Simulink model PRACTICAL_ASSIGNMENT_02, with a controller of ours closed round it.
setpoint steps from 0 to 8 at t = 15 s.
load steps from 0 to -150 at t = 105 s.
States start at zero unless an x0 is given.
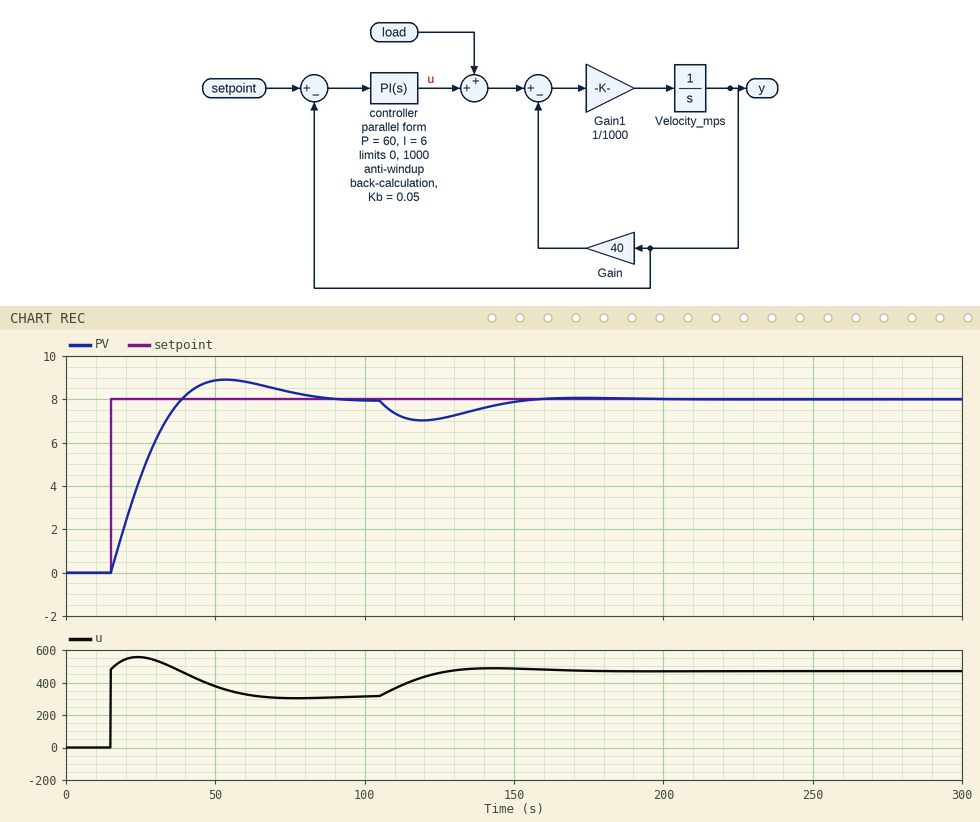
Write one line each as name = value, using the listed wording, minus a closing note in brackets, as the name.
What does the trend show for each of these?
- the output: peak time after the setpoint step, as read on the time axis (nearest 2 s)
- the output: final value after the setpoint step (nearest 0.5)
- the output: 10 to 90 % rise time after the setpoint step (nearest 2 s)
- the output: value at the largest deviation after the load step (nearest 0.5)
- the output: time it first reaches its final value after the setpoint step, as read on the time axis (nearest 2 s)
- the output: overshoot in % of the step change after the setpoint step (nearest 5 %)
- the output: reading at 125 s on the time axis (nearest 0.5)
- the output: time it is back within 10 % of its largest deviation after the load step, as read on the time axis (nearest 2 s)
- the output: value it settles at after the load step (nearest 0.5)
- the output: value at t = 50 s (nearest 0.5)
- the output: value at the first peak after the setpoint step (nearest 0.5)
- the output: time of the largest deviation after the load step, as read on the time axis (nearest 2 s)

the output: peak time after the setpoint step, as read on the time axis = 54 s
the output: final value after the setpoint step = 8.0
the output: 10 to 90 % rise time after the setpoint step = 18 s
the output: value at the largest deviation after the load step = 7.0
the output: time it first reaches its final value after the setpoint step, as read on the time axis = 38 s
the output: overshoot in % of the step change after the setpoint step = 10 %
the output: reading at 125 s on the time axis = 7.0
the output: time it is back within 10 % of its largest deviation after the load step, as read on the time axis = 152 s
the output: value it settles at after the load step = 8.0
the output: value at t = 50 s = 9.0
the output: value at the first peak after the setpoint step = 9.0
the output: time of the largest deviation after the load step, as read on the time axis = 120 s
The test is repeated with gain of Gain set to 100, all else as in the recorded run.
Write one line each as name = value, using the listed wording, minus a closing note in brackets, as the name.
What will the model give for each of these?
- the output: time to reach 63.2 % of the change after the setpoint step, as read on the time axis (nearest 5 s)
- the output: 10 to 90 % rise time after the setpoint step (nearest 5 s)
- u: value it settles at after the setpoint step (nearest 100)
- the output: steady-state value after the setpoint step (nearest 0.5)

the output: time to reach 63.2 % of the change after the setpoint step, as read on the time axis = 30 s
the output: 10 to 90 % rise time after the setpoint step = 35 s
u: value it settles at after the setpoint step = 800
the output: steady-state value after the setpoint step = 8.0
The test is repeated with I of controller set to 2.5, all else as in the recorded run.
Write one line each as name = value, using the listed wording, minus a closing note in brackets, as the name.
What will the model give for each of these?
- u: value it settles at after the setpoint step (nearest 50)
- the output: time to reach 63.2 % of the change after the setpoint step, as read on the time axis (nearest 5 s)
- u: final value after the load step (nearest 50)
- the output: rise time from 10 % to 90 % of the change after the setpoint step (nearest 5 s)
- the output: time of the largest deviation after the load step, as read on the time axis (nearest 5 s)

u: value it settles at after the setpoint step = 300
the output: time to reach 63.2 % of the change after the setpoint step, as read on the time axis = 30 s
u: final value after the load step = 450
the output: rise time from 10 % to 90 % of the change after the setpoint step = 35 s
the output: time of the largest deviation after the load step, as read on the time axis = 125 s
